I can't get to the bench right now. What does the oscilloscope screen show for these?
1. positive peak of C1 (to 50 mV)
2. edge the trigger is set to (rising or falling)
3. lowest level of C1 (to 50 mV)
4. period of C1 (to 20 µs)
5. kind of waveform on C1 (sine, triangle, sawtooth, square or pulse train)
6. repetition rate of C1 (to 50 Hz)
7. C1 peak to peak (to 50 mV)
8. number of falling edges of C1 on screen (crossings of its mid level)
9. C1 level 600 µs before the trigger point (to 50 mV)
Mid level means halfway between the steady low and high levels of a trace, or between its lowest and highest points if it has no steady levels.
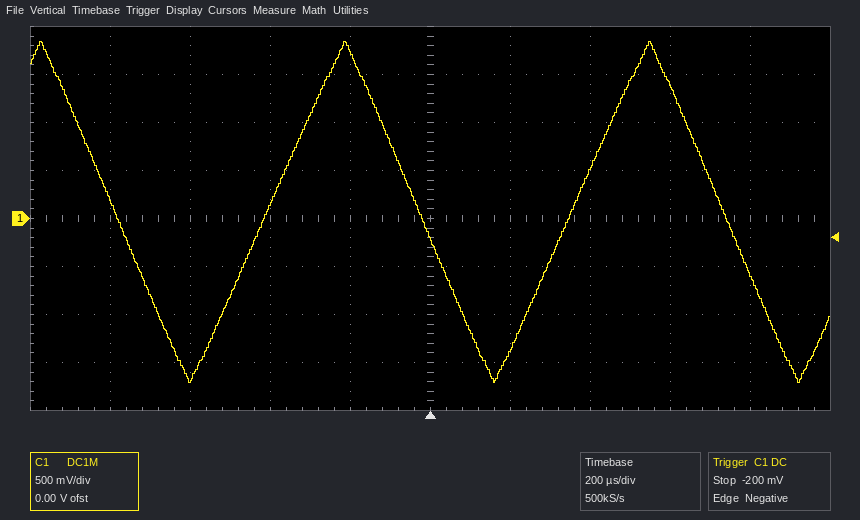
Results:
1.85 V
falling
-1.70 V
760 µs
triangle
1.30 kHz
3.55 V
3
-1.65 V
